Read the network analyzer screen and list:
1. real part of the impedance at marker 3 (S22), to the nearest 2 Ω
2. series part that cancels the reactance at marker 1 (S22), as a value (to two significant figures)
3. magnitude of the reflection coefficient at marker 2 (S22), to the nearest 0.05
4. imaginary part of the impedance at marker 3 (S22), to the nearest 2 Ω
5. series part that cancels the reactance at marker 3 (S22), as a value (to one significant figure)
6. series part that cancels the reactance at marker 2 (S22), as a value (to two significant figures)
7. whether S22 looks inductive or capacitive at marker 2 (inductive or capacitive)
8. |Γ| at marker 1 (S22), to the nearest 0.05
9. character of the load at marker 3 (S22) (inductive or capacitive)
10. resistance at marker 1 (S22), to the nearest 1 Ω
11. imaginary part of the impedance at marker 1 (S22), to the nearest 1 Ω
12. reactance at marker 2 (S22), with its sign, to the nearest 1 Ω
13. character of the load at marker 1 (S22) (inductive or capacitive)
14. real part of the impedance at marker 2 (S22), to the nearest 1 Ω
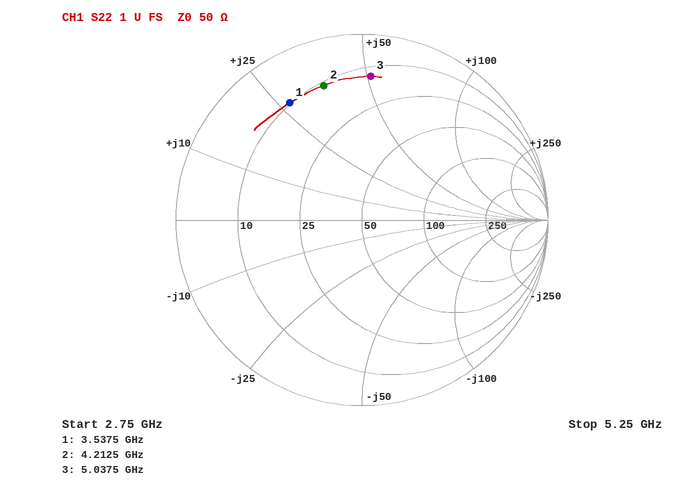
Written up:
14 Ω
1.7 pF
0.75
+52 Ω
600 fF
1.0 pF
inductive
0.75
inductive
10 Ω
+27 Ω
+37 Ω
inductive
11 Ω
